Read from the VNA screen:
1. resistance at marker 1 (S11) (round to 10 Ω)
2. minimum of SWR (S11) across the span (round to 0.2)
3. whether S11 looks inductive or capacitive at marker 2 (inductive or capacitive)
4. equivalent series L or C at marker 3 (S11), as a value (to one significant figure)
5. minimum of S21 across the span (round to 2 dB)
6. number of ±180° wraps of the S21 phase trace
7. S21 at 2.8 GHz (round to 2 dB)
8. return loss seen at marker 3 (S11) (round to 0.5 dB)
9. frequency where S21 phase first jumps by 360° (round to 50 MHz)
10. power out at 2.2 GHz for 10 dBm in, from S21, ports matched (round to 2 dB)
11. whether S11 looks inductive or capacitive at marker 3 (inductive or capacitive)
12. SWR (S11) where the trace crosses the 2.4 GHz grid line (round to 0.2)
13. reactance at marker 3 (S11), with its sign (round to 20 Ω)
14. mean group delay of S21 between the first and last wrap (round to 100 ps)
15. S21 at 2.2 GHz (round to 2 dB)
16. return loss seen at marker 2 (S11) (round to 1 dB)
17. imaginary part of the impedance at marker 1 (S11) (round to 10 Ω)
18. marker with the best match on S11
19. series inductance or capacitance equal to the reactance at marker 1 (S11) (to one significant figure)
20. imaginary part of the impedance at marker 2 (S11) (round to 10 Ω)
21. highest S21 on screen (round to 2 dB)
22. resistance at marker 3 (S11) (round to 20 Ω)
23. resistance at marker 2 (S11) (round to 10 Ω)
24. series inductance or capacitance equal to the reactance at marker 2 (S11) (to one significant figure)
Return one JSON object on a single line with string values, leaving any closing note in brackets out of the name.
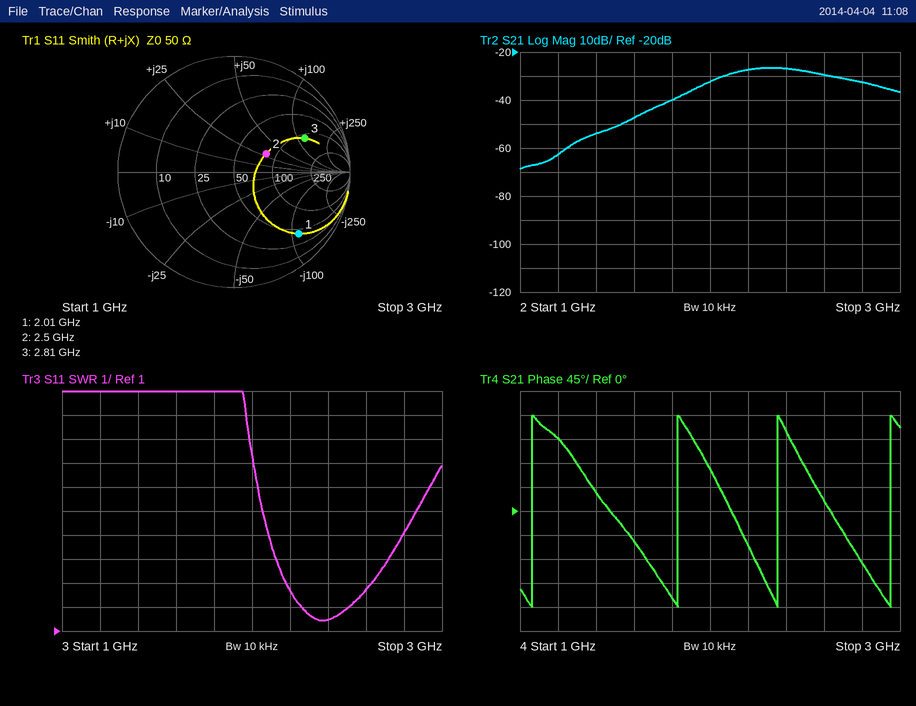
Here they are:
{"resistance at marker 1 (S11)": "40 Ω", "minimum of SWR (S11) across the span": "1.4", "whether S11 looks inductive or capacitive at marker 2": "inductive", "equivalent series L or C at marker 3 (S11), as a value": "7 nH", "minimum of S21 across the span": "-68 dB", "number of ±180° wraps of the S21 phase trace": "4", "S21 at 2.8 GHz": "-32 dB", "return loss seen at marker 3 (S11)": "3.5 dB", "frequency where S21 phase first jumps by 360°": "1.05 GHz", "power out at 2.2 GHz for 10 dBm in, from S21, ports matched": "-18 dBm", "whether S11 looks inductive or capacitive at marker 3": "inductive", "SWR (S11) where the trace crosses the 2.4 GHz grid line": "1.4", "reactance at marker 3 (S11), with its sign": "+120 Ω", "mean group delay of S21 between the first and last wrap": "1.6 ns", "S21 at 2.2 GHz": "-28 dB", "return loss seen at marker 2 (S11)": "10 dB", "imaginary part of the impedance at marker 1 (S11)": "-110 Ω", "marker with the best match on S11": "marker 2", "series inductance or capacitance equal to the reactance at marker 1 (S11)": "700 fF", "imaginary part of the impedance at marker 2 (S11)": "+30 Ω", "highest S21 on screen": "-26 dB", "resistance at marker 3 (S11)": "120 Ω", "resistance at marker 2 (S11)": "80 Ω", "series inductance or capacitance equal to the reactance at marker 2 (S11)": "2 nH"}
